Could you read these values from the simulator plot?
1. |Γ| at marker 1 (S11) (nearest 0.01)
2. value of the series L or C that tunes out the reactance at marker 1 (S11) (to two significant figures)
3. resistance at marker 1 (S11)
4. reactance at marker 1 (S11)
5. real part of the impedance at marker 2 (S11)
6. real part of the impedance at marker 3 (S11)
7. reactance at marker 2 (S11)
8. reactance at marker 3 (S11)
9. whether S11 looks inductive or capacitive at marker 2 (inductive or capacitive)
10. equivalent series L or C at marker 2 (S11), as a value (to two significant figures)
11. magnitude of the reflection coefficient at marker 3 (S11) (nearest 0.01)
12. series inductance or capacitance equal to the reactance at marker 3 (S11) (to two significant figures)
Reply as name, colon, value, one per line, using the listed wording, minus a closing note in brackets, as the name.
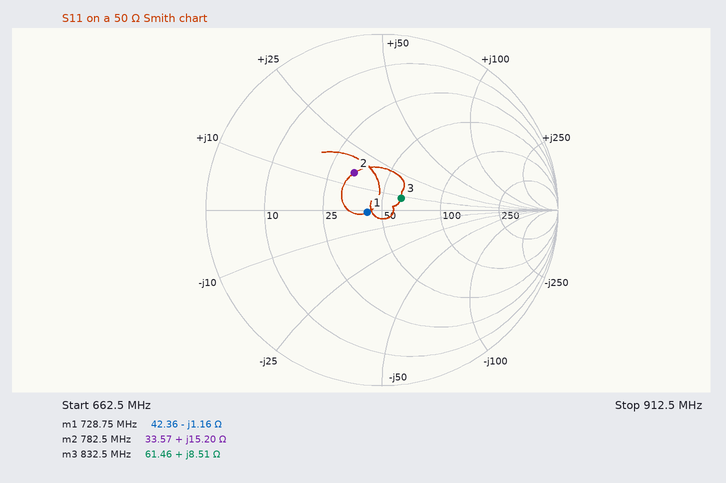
|Γ| at marker 1 (S11): 0.08
value of the series L or C that tunes out the reactance at marker 1 (S11): 250 pH
resistance at marker 1: 42.36 Ω
reactance at marker 1: -1.16 Ω
real part of the impedance at marker 2: 33.57 Ω
real part of the impedance at marker 3: 61.46 Ω
reactance at marker 2: +15.20 Ω
reactance at marker 3: +8.51 Ω
whether S11 looks inductive or capacitive at marker 2: inductive
equivalent series L or C at marker 2 (S11), as a value: 3.1 nH
magnitude of the reflection coefficient at marker 3 (S11): 0.13
series inductance or capacitance equal to the reactance at marker 3 (S11): 1.6 nH
